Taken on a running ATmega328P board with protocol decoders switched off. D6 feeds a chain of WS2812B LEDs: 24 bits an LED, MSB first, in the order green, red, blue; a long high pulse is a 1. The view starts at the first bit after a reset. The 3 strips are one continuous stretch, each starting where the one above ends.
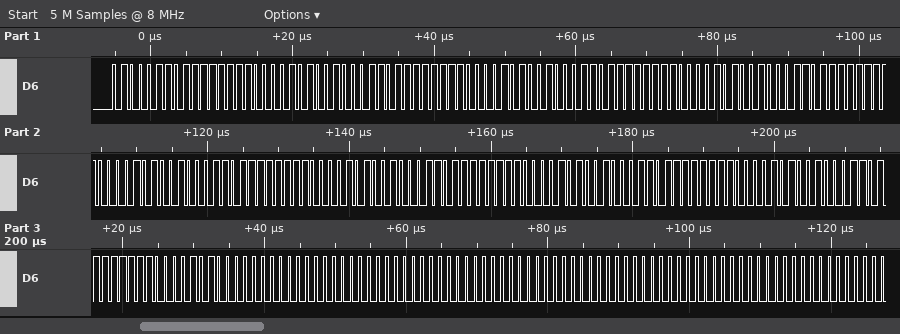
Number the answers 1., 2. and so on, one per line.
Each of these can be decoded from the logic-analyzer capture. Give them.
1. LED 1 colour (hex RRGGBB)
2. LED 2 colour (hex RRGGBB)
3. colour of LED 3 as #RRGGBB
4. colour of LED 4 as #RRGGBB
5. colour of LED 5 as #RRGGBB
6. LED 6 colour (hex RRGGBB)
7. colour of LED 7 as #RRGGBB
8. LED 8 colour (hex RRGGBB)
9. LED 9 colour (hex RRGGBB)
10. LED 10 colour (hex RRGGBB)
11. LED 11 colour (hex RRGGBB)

1. #FF460A
2. #FF460A
3. #FF460A
4. #FF460A
5. #FF460A
6. #FF460A
7. #FF460A
8. #FF460A
9. #000000
10. #000000
11. #000000
